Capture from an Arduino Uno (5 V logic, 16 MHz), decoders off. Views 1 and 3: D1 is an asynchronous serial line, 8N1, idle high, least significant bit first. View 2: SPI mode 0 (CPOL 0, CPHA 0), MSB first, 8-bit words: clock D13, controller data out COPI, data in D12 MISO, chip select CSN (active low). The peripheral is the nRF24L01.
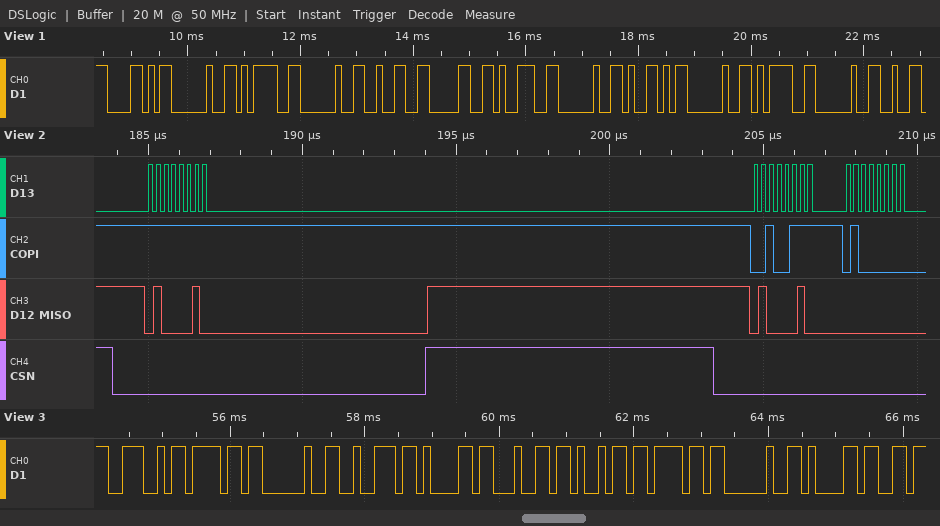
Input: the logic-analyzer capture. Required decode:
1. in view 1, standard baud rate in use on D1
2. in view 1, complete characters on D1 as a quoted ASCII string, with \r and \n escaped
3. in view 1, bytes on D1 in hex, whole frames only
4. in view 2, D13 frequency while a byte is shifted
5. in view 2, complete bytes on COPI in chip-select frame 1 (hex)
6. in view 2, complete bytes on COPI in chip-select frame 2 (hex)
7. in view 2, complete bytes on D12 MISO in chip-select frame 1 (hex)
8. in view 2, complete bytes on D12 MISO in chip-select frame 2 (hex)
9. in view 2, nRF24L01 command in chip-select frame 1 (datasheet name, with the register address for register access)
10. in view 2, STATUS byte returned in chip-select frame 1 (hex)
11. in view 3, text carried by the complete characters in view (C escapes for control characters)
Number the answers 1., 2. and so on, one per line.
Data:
1. 9600 baud
2. "X = 209 Y = "
3. 0x58 0x20 0x3D 0x20 0x32 0x30 0x39 0x20 0x59 0x20 0x3D 0x20
4. 4 MHz
5. FF
6. 27 40
7. 42
8. 42 00
9. NOP
10. 0x42
11. "No radio a"
